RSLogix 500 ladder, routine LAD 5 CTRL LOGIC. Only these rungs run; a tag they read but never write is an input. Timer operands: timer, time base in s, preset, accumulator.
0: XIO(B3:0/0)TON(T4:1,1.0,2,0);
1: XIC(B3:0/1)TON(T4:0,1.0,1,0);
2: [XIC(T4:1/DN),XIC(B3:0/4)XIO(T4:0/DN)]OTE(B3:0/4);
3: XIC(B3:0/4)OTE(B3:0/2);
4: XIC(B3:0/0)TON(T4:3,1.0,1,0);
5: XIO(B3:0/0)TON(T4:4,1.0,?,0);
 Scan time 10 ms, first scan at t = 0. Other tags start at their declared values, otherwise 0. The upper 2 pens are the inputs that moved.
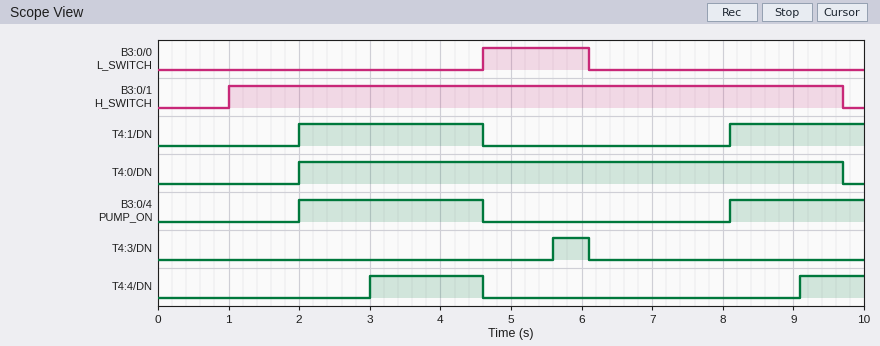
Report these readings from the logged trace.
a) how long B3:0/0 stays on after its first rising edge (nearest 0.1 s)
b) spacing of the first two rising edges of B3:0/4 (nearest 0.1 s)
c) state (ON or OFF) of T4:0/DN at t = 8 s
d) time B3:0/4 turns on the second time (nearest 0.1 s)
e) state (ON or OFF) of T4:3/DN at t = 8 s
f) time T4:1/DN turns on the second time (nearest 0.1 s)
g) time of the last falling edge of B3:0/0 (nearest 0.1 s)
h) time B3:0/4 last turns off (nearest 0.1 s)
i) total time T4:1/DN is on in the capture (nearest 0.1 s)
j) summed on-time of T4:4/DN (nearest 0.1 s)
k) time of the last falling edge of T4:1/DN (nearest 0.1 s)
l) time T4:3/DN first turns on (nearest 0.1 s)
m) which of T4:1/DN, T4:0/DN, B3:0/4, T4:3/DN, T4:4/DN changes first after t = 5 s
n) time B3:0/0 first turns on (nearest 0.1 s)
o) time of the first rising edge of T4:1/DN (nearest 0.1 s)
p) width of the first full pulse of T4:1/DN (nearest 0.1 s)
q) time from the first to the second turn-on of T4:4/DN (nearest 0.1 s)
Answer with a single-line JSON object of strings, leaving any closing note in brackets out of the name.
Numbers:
{"how long B3:0/0 stays on after its first rising edge": "1.5 s", "spacing of the first two rising edges of B3:0/4": "6.1 s", "state (ON or OFF) of T4:0/DN at t = 8 s": "ON", "time B3:0/4 turns on the second time": "8.1 s", "state (ON or OFF) of T4:3/DN at t = 8 s": "OFF", "time T4:1/DN turns on the second time": "8.1 s", "time of the last falling edge of B3:0/0": "6.1 s", "time B3:0/4 last turns off": "4.6 s", "total time T4:1/DN is on in the capture": "4.5 s", "summed on-time of T4:4/DN": "2.5 s", "time of the last falling edge of T4:1/DN": "4.6 s", "time T4:3/DN first turns on": "5.6 s", "which of T4:1/DN, T4:0/DN, B3:0/4, T4:3/DN, T4:4/DN changes first after t = 5 s": "T4:3/DN", "time B3:0/0 first turns on": "4.6 s", "time of the first rising edge of T4:1/DN": "2.0 s", "width of the first full pulse of T4:1/DN": "2.6 s", "time from the first to the second turn-on of T4:4/DN": "6.1 s"}
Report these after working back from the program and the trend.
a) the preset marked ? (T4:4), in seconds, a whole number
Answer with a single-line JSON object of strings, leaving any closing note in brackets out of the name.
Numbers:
{"the preset marked ? (T4:4), in seconds, a whole number": "3 s"}
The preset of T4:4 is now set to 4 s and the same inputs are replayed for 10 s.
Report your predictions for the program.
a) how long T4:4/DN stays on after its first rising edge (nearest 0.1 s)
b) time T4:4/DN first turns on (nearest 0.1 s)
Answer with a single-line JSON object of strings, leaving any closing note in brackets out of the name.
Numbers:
{"how long T4:4/DN stays on after its first rising edge": "0.6 s", "time T4:4/DN first turns on": "4.0 s"}
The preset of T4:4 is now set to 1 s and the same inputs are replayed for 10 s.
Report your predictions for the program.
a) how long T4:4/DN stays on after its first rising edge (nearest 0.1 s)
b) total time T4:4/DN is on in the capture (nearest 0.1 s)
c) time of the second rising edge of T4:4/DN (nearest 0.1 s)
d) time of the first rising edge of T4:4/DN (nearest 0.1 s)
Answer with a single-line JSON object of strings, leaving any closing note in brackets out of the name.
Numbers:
{"how long T4:4/DN stays on after its first rising edge": "3.6 s", "total time T4:4/DN is on in the capture": "6.5 s", "time of the second rising edge of T4:4/DN": "7.1 s", "time of the first rising edge of T4:4/DN": "1.0 s"}
